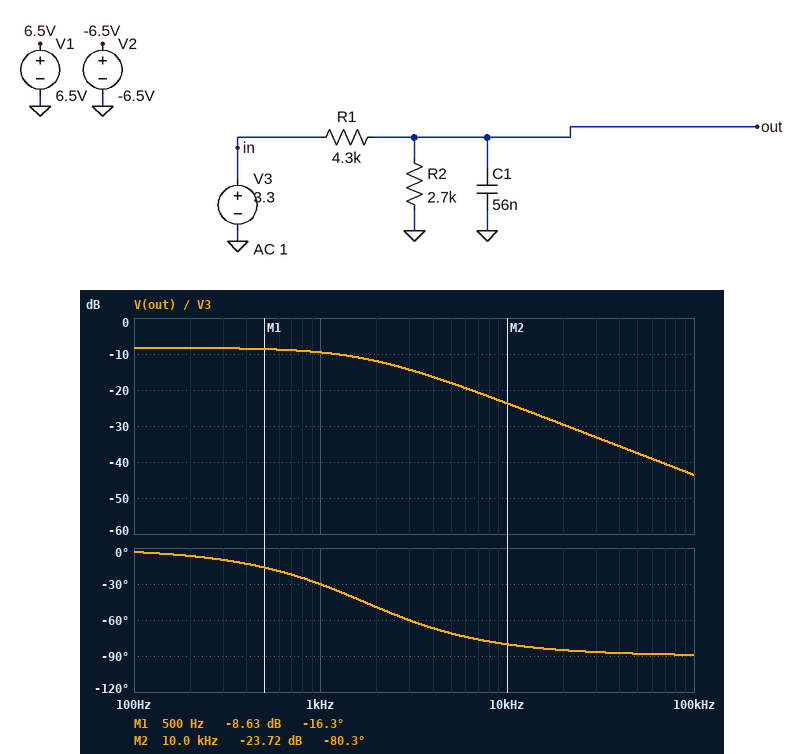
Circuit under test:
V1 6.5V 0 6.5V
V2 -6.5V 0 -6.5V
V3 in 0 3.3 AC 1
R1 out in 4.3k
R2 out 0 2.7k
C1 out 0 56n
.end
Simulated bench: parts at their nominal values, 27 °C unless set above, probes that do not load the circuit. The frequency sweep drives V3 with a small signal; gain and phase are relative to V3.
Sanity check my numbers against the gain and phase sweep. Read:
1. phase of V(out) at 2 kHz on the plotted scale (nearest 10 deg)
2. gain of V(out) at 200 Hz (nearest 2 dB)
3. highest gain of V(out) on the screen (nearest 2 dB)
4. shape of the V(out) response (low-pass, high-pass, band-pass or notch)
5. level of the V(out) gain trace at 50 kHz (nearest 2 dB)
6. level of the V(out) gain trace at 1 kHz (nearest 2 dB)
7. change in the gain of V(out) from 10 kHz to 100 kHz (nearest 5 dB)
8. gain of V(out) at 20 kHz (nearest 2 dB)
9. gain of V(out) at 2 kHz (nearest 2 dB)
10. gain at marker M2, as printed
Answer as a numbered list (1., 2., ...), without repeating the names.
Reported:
1. -50 deg
2. -8 dB
3. -8 dB
4. low-pass
5. -38 dB
6. -10 dB
7. -20 dB
8. -30 dB
9. -12 dB
10. -23.72 dB
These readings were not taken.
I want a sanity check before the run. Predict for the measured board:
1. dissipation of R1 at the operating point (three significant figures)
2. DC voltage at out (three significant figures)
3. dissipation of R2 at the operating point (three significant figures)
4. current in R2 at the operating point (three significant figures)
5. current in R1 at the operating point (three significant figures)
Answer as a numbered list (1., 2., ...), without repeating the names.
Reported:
1. 956 µW
2. 1.27 V
3. 600 µW
4. 471 µA
5. 471 µA
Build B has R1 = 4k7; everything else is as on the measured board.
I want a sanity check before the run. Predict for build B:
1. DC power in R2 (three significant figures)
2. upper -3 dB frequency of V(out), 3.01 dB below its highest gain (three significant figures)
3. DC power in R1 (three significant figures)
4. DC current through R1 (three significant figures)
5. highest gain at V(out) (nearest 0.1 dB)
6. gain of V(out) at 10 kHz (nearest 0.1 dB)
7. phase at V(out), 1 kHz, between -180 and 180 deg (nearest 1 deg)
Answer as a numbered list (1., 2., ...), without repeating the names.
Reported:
1. 537 µW
2. 1.66 kHz
3. 935 µW
4. 446 µA
5. -8.8 dB
6. -24.5 dB
7. -31 deg
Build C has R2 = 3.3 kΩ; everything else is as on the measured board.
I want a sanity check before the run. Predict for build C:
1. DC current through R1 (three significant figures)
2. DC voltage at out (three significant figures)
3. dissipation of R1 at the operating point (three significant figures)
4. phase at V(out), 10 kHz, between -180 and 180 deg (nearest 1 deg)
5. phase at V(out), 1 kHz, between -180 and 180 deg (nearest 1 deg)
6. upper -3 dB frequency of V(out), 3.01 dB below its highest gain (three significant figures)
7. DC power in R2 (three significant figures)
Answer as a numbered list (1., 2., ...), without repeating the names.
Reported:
1. 434 µA
2. 1.43 V
3. 811 µW
4. -81 deg
5. -33 deg
6. 1.52 kHz
7. 622 µW
